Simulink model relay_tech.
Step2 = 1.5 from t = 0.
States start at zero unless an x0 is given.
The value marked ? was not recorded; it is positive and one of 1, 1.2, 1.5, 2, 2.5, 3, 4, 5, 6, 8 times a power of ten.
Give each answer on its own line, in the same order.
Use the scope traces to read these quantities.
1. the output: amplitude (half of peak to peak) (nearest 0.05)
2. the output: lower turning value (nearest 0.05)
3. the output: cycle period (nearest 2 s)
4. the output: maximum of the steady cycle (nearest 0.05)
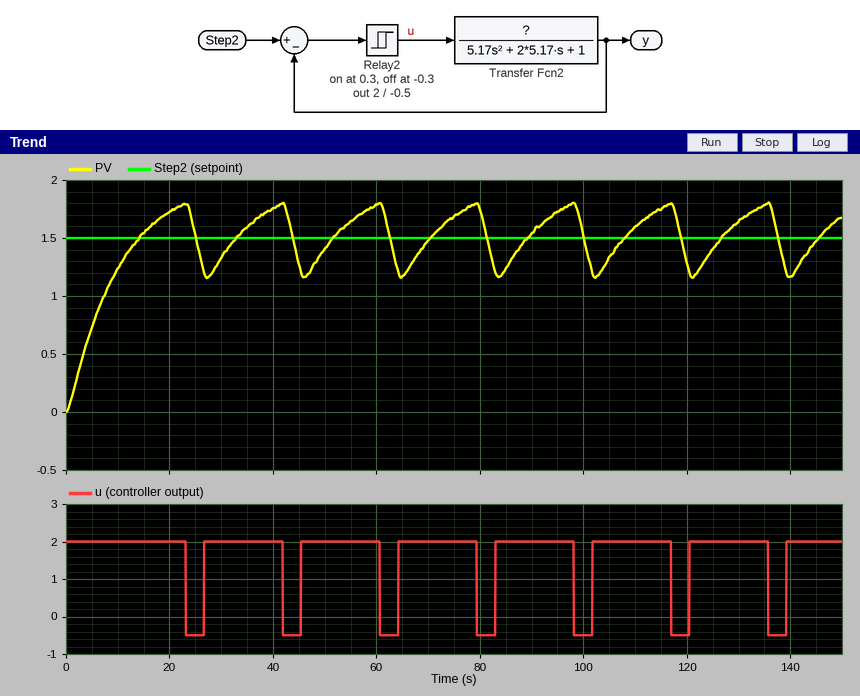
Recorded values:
0.30
1.15
18 s
1.80
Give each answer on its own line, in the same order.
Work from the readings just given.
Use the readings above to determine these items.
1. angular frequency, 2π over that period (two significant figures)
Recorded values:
0.35 rad/s
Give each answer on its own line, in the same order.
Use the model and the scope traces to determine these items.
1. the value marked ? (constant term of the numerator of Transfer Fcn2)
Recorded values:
1
